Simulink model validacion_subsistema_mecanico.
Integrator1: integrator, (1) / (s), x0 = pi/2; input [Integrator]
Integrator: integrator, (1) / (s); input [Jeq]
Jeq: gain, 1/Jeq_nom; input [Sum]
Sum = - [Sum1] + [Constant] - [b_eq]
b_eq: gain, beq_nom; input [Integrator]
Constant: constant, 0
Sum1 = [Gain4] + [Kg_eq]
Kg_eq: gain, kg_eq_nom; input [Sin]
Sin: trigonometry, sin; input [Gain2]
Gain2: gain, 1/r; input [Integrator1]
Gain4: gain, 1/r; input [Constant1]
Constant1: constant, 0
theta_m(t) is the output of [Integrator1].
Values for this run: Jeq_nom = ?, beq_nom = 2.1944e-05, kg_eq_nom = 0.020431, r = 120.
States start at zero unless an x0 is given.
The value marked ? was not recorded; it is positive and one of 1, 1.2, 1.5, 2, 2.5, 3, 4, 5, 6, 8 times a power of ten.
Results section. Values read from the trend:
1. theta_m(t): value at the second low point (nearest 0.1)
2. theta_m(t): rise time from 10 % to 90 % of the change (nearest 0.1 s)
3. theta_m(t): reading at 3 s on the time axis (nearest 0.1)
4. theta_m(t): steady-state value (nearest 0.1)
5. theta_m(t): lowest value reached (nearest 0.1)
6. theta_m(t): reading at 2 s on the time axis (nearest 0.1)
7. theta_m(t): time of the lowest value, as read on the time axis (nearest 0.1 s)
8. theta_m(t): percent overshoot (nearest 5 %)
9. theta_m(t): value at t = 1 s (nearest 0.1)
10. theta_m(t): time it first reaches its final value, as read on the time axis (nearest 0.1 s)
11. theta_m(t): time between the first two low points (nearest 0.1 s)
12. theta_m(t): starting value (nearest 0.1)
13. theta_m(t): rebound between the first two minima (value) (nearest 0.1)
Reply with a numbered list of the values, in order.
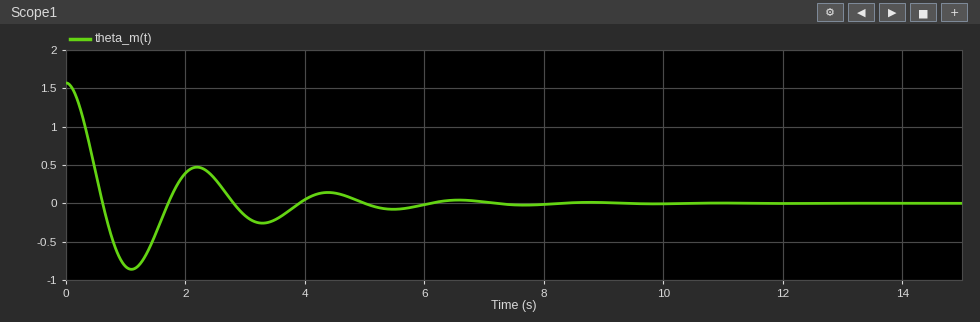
1. -0.3
2. 0.4 s
3. -0.2
4. 0.0
5. -0.9
6. 0.4
7. 1.1 s
8. 55 %
9. -0.8
10. 0.6 s
11. 2.2 s
12. 1.6
13. 0.5
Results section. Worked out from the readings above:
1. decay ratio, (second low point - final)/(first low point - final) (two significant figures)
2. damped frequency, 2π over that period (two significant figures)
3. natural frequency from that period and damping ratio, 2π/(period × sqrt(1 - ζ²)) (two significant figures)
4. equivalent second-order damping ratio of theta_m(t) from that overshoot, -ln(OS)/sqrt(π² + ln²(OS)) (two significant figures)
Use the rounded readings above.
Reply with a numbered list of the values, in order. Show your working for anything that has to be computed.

1. (-0.3 - 0) / (-0.9 - 0) = 0.33
2. 2π / 2.2 = 2.9 rad/s
3. 2π / (2.2 × sqrt(1 - 0.19²)) = 2.9 rad/s
4. ln(0.55) = -0.598; 0.598 / sqrt(9.870 + 0.357) = 0.19
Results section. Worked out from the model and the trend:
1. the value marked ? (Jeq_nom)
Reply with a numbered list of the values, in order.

1. 2e-05
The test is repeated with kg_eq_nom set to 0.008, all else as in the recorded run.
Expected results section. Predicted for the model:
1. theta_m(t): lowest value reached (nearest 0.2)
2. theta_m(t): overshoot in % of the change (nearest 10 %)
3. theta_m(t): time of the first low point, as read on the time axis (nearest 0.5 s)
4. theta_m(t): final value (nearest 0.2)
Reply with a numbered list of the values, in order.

1. -0.6
2. 40 %
3. 2.0 s
4. 0.0
